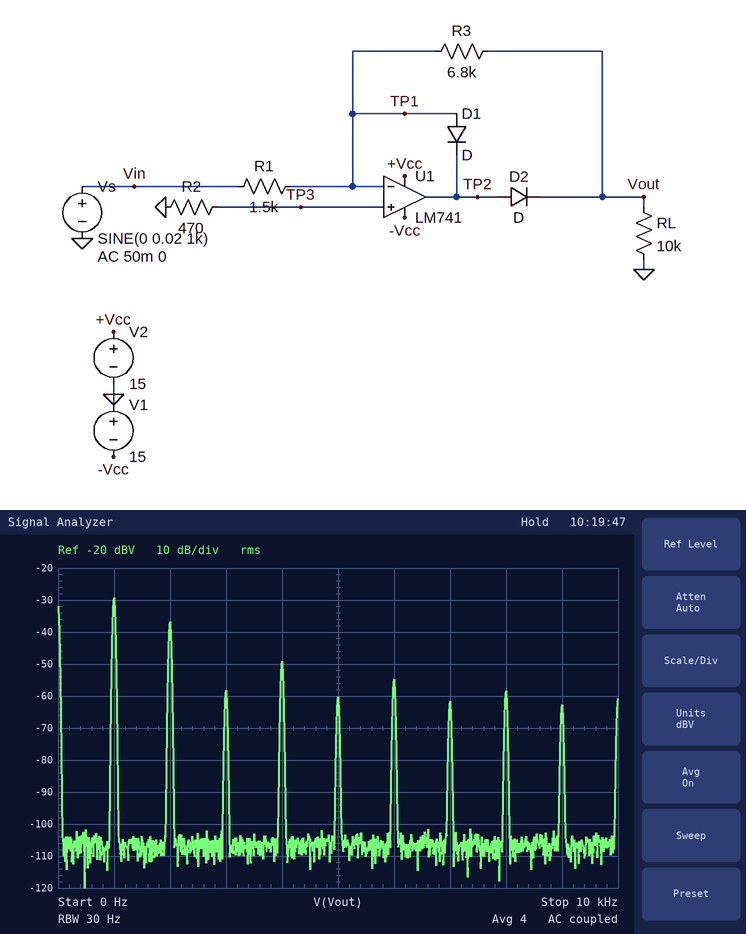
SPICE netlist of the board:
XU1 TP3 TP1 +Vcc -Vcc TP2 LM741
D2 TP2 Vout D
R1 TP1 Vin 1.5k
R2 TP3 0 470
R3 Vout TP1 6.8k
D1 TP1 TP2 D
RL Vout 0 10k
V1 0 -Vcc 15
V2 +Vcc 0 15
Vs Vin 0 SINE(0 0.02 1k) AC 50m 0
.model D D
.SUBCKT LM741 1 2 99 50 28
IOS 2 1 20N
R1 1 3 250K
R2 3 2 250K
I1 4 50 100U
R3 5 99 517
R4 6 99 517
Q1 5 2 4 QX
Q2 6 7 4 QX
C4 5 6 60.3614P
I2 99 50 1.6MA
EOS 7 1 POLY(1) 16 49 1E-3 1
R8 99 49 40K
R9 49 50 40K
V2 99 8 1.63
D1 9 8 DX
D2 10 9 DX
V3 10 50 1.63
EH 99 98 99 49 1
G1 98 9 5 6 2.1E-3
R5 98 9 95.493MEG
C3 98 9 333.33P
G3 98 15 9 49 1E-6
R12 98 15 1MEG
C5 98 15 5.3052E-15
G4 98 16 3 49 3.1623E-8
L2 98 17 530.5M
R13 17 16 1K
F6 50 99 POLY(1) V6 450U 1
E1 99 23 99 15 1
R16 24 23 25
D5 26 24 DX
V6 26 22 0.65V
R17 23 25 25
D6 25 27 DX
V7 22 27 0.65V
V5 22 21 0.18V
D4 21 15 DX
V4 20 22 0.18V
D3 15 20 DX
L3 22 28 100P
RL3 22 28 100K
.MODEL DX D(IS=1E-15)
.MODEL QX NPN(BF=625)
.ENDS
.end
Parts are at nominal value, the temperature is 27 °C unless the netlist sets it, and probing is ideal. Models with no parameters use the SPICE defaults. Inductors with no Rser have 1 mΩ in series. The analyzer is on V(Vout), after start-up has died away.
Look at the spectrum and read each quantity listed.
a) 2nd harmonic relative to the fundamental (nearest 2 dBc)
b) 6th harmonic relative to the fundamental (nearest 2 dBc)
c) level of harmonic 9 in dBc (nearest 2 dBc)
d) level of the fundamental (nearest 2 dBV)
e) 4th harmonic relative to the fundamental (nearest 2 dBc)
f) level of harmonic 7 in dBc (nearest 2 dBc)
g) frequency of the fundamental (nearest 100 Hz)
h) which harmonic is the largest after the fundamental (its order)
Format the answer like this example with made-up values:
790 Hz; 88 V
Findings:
-8 dBc; -26 dBc; -34 dBc; -30 dBV; -20 dBc; -32 dBc; 1.0 kHz; 2
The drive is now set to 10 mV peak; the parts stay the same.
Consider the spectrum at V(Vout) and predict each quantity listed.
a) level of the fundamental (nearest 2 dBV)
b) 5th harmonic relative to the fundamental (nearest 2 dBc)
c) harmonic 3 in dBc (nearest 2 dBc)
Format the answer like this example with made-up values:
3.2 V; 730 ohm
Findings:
-34 dBV; -28 dBc; -24 dBc
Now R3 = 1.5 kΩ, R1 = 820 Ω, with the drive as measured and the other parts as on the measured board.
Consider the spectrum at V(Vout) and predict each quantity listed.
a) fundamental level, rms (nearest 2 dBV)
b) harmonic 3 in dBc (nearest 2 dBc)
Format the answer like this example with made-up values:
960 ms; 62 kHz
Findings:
-38 dBV; -26 dBc
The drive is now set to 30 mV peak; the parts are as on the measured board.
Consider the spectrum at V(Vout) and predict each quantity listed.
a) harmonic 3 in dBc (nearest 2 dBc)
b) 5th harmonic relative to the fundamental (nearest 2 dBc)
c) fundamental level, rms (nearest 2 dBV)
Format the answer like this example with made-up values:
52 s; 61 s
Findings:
-32 dBc; -34 dBc; -26 dBV
